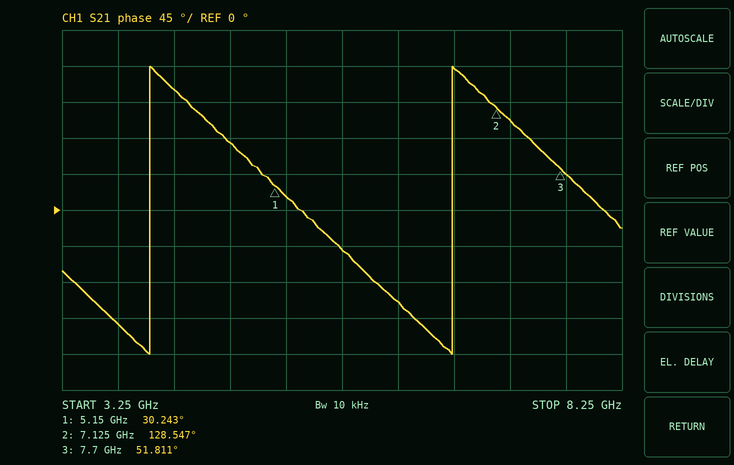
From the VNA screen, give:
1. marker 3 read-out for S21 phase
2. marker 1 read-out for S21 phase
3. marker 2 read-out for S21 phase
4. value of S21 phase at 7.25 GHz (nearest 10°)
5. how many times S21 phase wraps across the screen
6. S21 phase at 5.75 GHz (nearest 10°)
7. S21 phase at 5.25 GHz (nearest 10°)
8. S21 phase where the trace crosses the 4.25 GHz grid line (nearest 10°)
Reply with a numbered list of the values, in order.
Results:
1. 51.811°
2. 30.243°
3. 128.547°
4. 110°
5. 2
6. -50°
7. 20°
8. 150°
